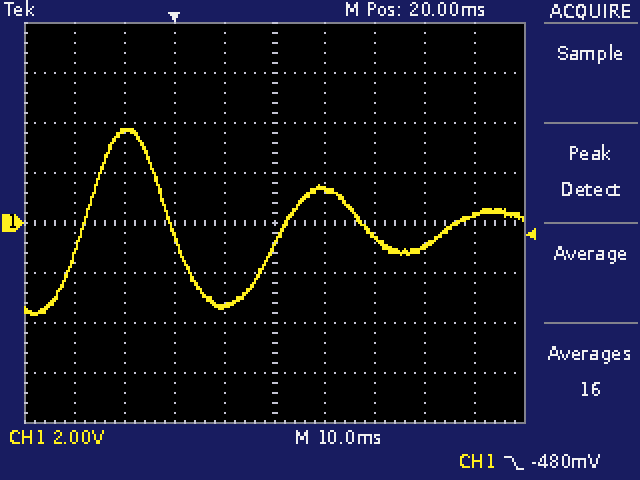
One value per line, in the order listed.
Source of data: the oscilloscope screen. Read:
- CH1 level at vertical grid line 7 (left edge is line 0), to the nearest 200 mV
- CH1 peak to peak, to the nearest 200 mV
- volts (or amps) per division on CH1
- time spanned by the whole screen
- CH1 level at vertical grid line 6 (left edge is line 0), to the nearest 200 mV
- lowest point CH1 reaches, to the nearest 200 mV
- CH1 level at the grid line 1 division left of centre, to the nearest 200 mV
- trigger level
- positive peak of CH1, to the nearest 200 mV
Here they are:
-600 mV
7.4 V
2 V
100 ms
1.4 V
-3.6 V
-3.4 V
-480 mV
3.8 V
